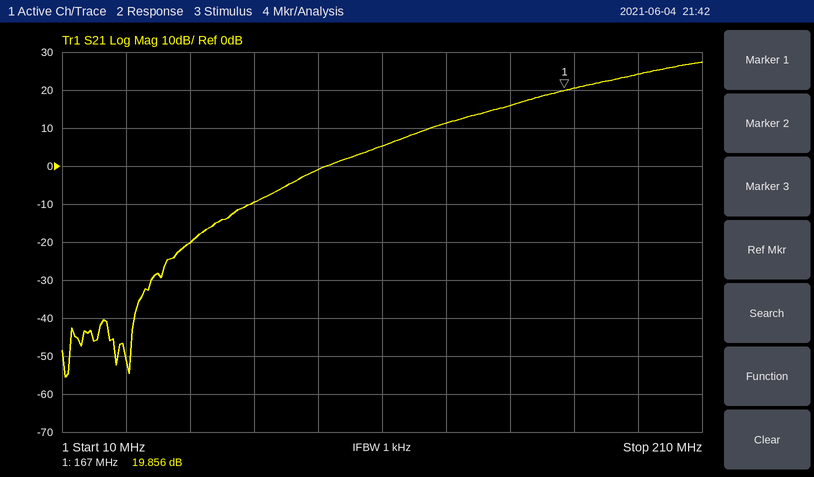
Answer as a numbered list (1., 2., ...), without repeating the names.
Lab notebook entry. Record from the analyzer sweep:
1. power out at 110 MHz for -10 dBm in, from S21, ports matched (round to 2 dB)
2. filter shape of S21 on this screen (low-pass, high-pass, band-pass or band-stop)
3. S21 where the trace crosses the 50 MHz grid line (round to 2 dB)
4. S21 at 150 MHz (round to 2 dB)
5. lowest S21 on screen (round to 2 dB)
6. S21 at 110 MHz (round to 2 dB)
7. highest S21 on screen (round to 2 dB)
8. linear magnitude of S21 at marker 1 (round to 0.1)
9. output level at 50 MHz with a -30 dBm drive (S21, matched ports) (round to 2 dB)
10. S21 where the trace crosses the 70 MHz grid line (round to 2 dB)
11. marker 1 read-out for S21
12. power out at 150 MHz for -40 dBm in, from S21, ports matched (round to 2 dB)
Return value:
1. -4 dBm
2. high-pass
3. -20 dB
4. 16 dB
5. -56 dB
6. 6 dB
7. 28 dB
8. 9.8
9. -50 dBm
10. -10 dB
11. 19.856 dB
12. -24 dBm
